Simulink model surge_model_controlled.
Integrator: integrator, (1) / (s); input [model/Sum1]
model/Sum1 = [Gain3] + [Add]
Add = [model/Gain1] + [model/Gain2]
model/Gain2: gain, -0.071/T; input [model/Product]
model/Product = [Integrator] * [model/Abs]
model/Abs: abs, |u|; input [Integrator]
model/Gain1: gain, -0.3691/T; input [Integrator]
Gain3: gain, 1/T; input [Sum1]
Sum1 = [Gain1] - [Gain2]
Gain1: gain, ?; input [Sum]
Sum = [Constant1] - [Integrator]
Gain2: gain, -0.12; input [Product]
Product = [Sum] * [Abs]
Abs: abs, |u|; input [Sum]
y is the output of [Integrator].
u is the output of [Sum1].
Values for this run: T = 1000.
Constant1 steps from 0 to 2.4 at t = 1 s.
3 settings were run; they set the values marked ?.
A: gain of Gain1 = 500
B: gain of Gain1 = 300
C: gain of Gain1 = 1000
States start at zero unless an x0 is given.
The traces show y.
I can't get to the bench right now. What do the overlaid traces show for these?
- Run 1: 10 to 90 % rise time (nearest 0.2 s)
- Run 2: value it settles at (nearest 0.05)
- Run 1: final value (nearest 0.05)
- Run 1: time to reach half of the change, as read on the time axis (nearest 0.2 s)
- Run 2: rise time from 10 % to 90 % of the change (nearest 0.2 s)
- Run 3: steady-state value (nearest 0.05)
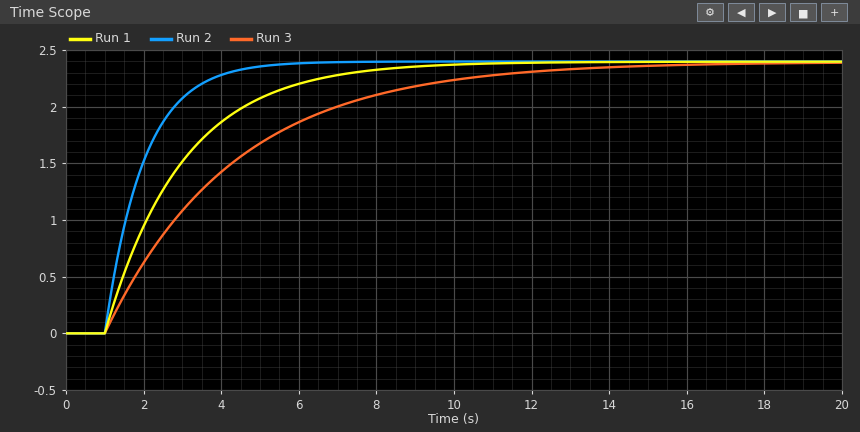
4.4 s
2.40
2.40
2.4 s
2.2 s
2.40
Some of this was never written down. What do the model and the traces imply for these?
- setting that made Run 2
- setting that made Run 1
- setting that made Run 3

C
A
B
